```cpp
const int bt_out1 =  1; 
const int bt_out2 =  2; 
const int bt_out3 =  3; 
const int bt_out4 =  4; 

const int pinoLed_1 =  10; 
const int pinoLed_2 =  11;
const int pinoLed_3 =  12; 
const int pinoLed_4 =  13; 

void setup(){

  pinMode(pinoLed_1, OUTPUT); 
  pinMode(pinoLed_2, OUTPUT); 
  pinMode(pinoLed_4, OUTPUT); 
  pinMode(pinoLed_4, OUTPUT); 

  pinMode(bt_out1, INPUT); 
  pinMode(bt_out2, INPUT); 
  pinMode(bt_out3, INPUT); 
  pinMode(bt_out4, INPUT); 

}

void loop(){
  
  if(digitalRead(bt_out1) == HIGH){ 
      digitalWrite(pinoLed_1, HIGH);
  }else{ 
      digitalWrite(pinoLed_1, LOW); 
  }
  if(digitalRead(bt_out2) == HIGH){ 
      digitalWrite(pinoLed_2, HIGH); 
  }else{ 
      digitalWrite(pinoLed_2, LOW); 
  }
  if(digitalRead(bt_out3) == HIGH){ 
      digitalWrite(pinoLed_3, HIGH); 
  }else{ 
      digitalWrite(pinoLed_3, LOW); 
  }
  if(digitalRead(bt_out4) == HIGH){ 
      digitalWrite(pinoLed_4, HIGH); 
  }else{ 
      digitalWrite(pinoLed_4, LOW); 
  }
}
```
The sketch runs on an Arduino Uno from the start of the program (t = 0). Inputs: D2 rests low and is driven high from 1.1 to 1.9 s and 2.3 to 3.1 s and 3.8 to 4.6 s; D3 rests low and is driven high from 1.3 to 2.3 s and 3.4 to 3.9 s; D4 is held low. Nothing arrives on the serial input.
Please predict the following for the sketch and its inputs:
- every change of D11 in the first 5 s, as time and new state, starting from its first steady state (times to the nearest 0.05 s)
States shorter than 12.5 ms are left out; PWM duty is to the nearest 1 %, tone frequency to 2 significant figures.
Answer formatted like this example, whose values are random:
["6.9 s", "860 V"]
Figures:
["0 s low; 1.1 s high; 1.9 s low; 2.3 s high; 3.1 s low; 3.8 s high; 4.6 s low"]
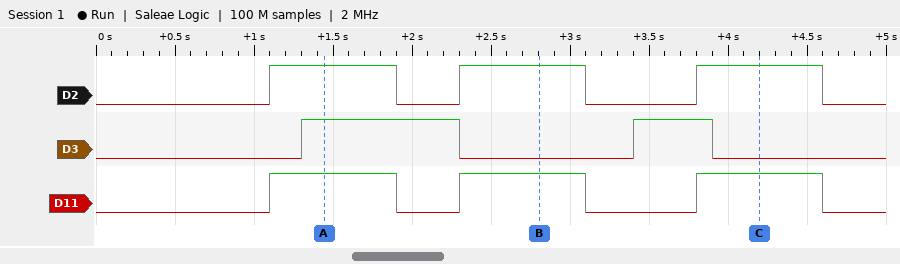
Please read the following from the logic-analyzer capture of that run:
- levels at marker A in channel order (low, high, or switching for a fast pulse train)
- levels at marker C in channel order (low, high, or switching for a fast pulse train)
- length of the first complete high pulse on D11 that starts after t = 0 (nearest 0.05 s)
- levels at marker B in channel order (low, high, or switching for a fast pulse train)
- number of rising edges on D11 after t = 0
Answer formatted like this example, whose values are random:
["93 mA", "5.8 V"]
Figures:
["D2 high, D3 high, D11 high", "D2 high, D3 low, D11 high", "0.80 s", "D2 high, D3 low, D11 high", "3"]
